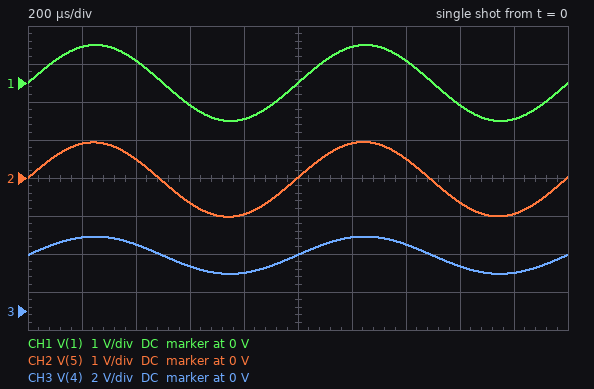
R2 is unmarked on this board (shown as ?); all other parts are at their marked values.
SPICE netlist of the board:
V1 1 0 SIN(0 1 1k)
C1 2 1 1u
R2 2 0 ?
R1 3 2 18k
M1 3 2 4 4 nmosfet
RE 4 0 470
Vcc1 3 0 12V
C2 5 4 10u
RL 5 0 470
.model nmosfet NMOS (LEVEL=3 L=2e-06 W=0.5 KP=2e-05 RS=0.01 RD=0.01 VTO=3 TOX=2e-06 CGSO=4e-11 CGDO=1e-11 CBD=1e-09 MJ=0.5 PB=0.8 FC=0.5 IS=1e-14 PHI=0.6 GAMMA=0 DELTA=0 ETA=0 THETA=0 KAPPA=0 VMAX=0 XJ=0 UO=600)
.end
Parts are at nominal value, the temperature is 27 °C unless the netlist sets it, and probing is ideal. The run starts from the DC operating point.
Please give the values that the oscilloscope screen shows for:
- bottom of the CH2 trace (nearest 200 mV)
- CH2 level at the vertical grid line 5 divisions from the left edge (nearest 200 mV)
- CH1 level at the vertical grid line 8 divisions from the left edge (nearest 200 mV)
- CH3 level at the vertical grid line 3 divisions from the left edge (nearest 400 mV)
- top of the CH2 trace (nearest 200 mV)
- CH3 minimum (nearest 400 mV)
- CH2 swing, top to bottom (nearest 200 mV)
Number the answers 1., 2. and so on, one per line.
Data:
1. -1.0 V
2. 0 V
3. -600 mV
4. 2.4 V
5. 1.0 V
6. 2.0 V
7. 2.0 V
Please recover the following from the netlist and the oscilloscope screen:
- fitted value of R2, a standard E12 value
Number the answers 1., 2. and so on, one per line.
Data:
1. 18 kΩ
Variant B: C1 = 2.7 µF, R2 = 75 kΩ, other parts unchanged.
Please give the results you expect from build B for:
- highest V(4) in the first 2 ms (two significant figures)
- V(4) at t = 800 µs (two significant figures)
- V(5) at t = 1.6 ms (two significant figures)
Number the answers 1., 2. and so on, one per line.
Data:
1. 7.6 V
2. 5.7 V
3. -640 mV
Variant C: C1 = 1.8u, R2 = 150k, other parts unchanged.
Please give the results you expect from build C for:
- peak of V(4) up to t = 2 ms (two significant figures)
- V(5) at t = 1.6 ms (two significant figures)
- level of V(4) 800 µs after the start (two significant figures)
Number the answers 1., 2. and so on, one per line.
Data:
1. 8.6 V
2. -640 mV
3. 6.7 V
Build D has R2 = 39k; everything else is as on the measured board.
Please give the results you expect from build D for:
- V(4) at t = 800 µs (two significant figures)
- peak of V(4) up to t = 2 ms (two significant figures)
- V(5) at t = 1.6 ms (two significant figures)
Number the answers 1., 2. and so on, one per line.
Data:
1. 4.2 V
2. 6.1 V
3. -650 mV
